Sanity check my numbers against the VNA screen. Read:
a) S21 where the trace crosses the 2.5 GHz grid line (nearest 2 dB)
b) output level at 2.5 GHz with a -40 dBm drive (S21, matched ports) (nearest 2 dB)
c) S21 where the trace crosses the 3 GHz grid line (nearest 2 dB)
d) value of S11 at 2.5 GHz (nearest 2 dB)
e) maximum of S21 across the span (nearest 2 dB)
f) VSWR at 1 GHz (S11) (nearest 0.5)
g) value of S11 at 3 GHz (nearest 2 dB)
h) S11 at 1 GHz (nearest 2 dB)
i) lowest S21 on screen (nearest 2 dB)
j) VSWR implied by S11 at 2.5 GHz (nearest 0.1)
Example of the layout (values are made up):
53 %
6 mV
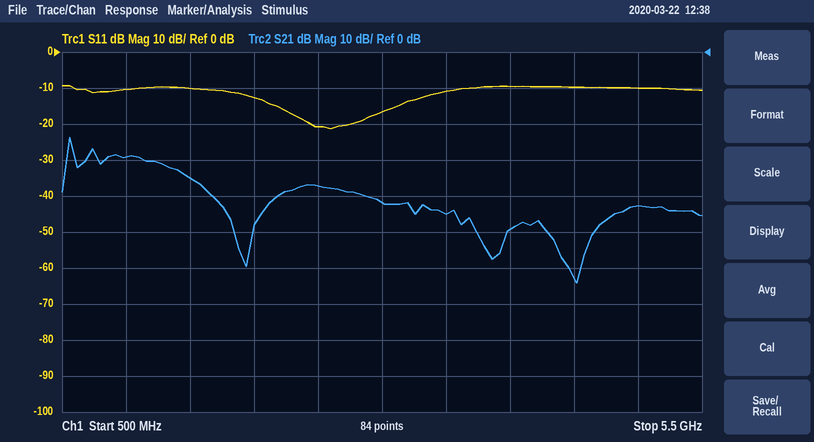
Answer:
-38 dB
-78 dBm
-42 dB
-20 dB
-24 dB
2.0
-16 dB
-10 dB
-64 dB
1.2
